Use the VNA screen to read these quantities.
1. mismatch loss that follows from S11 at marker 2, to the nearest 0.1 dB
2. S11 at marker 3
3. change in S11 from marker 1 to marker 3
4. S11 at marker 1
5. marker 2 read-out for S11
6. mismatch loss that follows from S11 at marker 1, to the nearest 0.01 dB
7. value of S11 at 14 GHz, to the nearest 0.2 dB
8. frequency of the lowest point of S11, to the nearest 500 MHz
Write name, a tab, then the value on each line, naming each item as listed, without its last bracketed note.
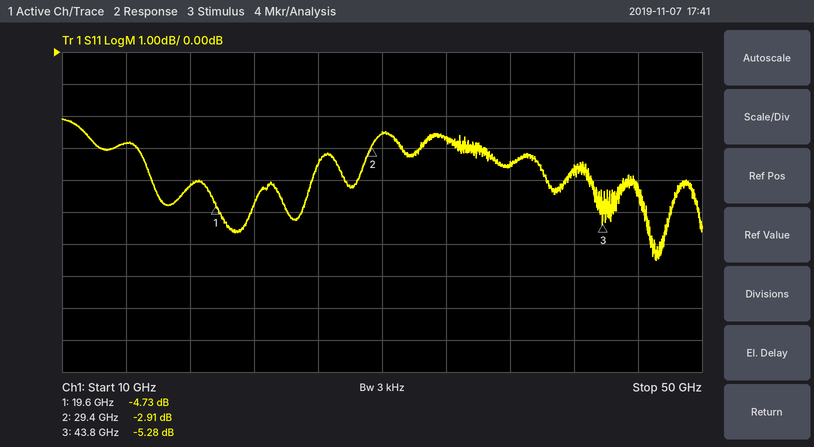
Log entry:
mismatch loss that follows from S11 at marker 2, to the nearest 0.1 dB	3.1 dB
S11 at marker 3	-5.28 dB
change in S11 from marker 1 to marker 3	-0.55 dB
S11 at marker 1	-4.73 dB
marker 2 read-out for S11	-2.91 dB
mismatch loss that follows from S11 at marker 1, to the nearest 0.01 dB	1.78 dB
value of S11 at 14 GHz, to the nearest 0.2 dB	-2.8 dB
frequency of the lowest point of S11, to the nearest 500 MHz	47.0 GHz
